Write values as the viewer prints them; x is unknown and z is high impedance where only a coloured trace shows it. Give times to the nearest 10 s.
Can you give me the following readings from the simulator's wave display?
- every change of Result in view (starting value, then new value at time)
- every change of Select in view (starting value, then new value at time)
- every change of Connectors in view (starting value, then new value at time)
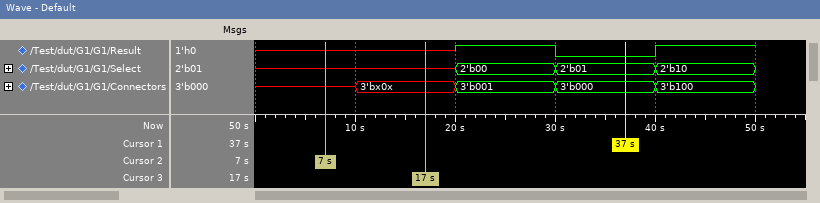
x, 1 at 20 s, 0 at 30 s, 1 at 40 s
x, 2'b00 at 20 s, 2'b01 at 30 s, 2'b10 at 40 s
x, 3'bx0x at 10 s, 3'b001 at 20 s, 3'b000 at 30 s, 3'b100 at 40 s
